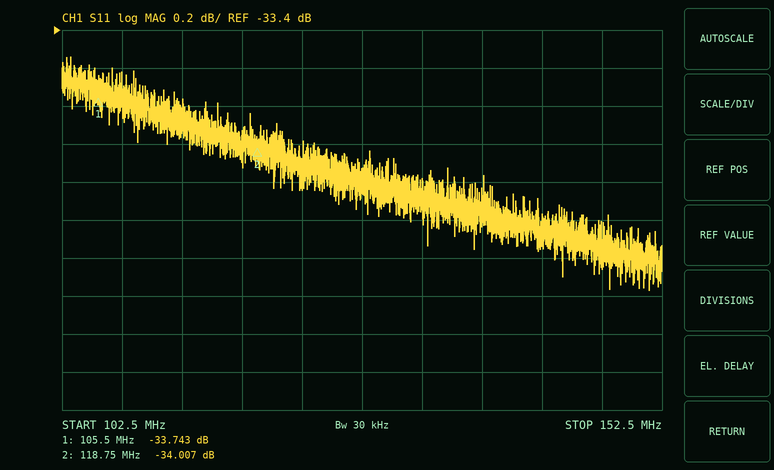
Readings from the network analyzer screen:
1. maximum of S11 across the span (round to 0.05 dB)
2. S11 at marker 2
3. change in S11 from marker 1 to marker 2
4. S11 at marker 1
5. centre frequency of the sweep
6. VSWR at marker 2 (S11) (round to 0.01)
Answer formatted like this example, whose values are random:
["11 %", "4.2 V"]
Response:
["-33.55 dB", "-34.007 dB", "-0.264 dB", "-33.743 dB", "127.5 MHz", "1.04"]
